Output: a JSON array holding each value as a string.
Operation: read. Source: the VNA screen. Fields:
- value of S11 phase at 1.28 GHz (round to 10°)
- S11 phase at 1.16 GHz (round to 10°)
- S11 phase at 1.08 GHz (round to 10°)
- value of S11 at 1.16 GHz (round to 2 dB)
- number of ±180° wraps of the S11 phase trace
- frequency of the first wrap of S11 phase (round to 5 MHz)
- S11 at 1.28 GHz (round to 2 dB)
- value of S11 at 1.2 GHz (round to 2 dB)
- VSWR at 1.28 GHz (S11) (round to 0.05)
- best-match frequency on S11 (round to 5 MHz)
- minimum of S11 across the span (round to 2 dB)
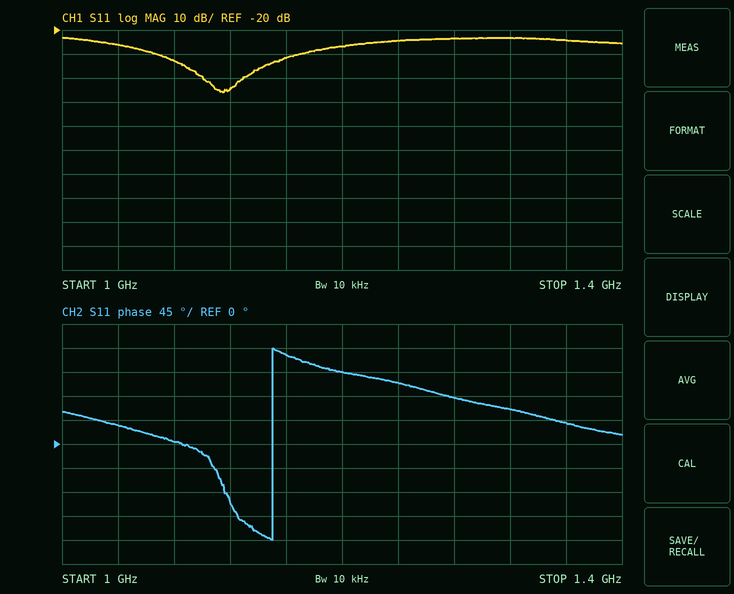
["90°", "170°", "0°", "-32 dB", "1", "1.150 GHz", "-24 dB", "-26 dB", "1.15", "1.115 GHz", "-46 dB"]
